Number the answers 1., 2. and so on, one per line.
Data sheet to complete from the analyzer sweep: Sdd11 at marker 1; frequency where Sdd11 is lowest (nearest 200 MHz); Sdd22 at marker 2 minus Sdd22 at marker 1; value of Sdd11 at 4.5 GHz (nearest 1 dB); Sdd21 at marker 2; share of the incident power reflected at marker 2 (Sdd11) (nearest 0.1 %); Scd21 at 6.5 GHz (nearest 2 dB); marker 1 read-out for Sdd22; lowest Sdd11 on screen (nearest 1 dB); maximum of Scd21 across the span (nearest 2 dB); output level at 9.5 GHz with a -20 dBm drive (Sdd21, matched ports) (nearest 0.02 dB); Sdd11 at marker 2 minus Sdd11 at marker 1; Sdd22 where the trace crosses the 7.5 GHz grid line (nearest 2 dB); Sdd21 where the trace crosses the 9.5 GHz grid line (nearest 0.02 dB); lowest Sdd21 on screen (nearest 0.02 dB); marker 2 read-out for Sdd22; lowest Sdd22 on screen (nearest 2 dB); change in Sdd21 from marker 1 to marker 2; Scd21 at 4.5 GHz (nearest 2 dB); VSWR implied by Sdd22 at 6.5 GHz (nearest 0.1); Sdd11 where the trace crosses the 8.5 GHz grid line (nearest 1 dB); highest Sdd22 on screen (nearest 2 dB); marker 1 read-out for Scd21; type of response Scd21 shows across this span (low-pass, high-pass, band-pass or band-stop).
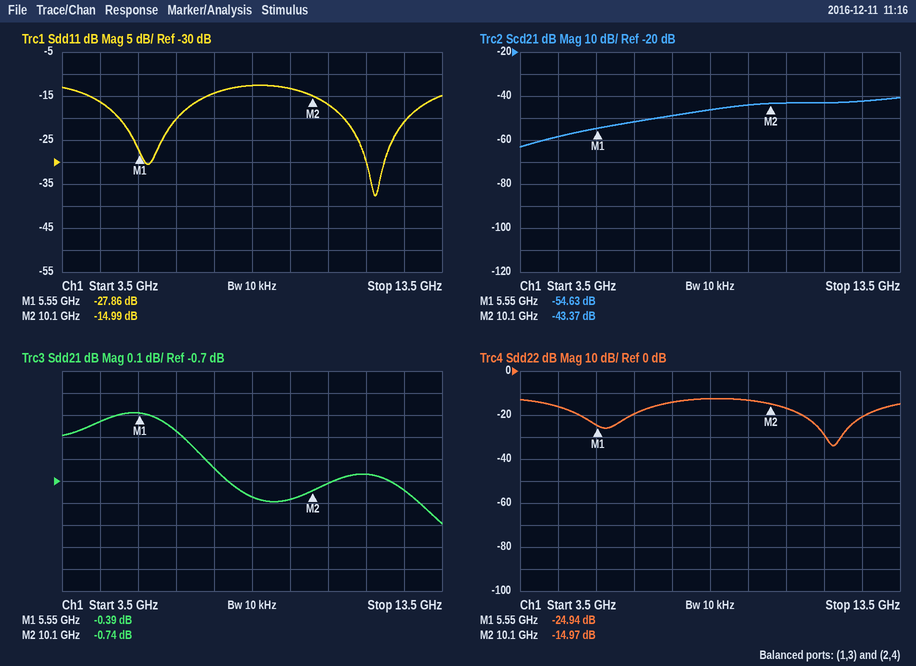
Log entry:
1. -27.86 dB
2. 11.8 GHz
3. 9.97 dB
4. -16 dB
5. -0.74 dB
6. 3.2 %
7. -52 dB
8. -24.94 dB
9. -38 dB
10. -40 dB
11. -20.78 dBm
12. 12.87 dB
13. -14 dB
14. -0.78 dB
15. -0.90 dB
16. -14.97 dB
17. -34 dB
18. -0.35 dB
19. -58 dB
20. 1.2
21. -13 dB
22. -12 dB
23. -54.63 dB
24. high-pass
